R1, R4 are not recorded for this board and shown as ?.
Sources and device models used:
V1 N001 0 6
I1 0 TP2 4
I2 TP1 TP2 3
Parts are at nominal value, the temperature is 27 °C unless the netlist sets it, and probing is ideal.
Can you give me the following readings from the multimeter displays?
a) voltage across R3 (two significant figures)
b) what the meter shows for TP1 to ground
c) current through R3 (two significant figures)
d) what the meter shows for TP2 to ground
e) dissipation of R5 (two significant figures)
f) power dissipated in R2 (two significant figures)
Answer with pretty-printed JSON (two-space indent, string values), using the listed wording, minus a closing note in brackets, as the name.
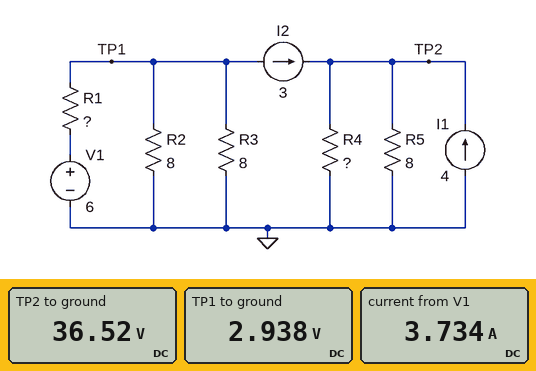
{
  "voltage across R3": "2.9 V",
  "what the meter shows for TP1 to ground": "2.938 V",
  "current through R3": "370 mA",
  "what the meter shows for TP2 to ground": "36.52 V",
  "dissipation of R5": "170 W",
  "power dissipated in R2": "1.1 W"
}
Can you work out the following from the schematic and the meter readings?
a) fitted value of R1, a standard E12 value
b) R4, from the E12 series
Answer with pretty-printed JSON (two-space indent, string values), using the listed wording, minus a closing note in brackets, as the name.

{
  "fitted value of R1, a standard E12 value": "0.82 Ω",
  "R4, from the E12 series": "15 Ω"
}
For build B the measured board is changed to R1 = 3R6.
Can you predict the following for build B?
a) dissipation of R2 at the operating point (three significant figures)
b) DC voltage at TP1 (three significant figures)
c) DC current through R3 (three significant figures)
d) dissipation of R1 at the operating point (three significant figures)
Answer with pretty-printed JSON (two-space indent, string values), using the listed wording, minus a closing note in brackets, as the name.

{
  "dissipation of R2 at the operating point": "798 mW",
  "DC voltage at TP1": "-2.53 V",
  "DC current through R3": "316 mA",
  "dissipation of R1 at the operating point": "20.2 W"
}
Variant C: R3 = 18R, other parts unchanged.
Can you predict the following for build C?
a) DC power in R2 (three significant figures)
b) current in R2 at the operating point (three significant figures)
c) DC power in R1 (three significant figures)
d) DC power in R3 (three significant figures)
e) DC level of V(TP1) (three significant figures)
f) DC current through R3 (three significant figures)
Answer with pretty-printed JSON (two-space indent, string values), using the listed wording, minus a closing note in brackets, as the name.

{
  "DC power in R2": "1.19 W",
  "current in R2 at the operating point": "385 mA",
  "DC power in R1": "10.4 W",
  "DC power in R3": "528 mW",
  "DC level of V(TP1)": "3.08 V",
  "DC current through R3": "171 mA"
}
